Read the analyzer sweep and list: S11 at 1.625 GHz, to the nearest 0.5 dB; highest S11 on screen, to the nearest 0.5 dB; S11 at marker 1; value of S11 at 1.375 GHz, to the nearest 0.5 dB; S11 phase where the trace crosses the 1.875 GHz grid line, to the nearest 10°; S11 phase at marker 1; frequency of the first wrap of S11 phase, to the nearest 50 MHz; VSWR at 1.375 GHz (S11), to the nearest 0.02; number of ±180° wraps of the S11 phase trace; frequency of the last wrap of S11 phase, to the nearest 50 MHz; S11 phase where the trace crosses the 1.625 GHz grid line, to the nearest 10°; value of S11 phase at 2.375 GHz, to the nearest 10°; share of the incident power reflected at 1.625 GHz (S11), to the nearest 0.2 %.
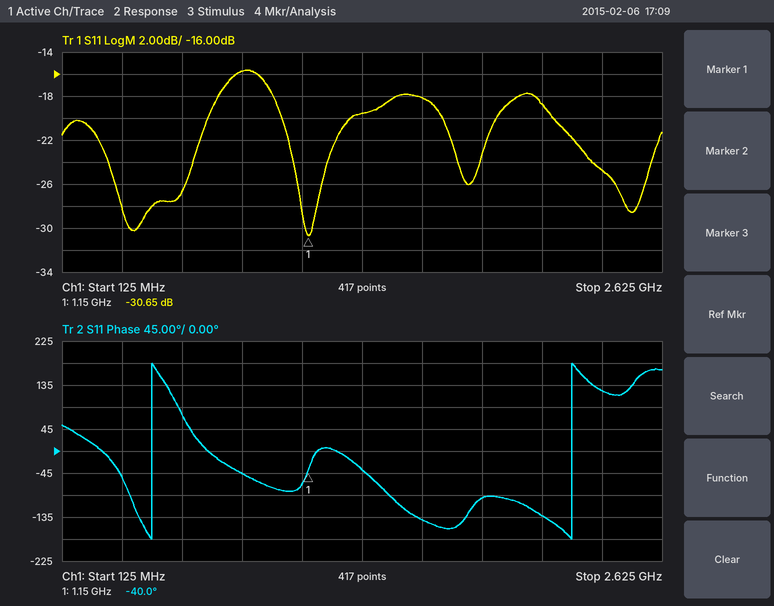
-18.0 dB
-15.5 dB
-30.65 dB
-19.5 dB
-100°
-40.0°
500 MHz
1.24
2
2.25 GHz
-140°
120°
1.6 %
